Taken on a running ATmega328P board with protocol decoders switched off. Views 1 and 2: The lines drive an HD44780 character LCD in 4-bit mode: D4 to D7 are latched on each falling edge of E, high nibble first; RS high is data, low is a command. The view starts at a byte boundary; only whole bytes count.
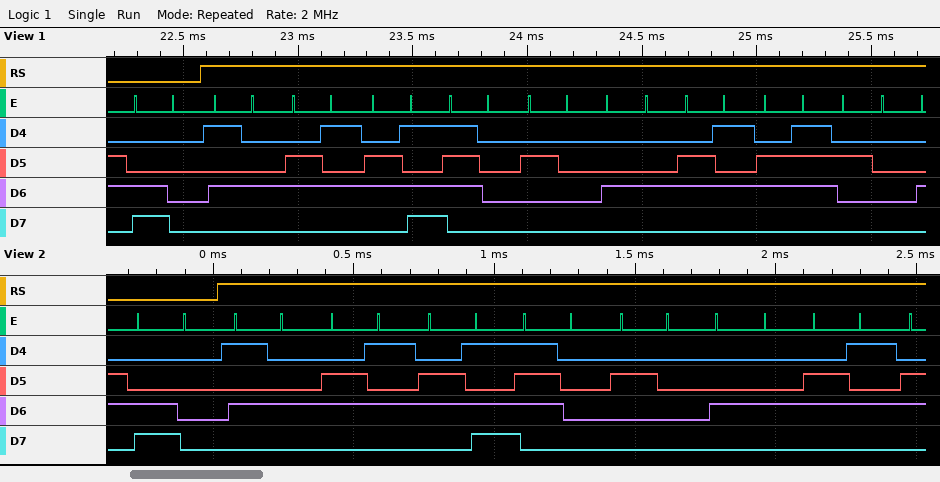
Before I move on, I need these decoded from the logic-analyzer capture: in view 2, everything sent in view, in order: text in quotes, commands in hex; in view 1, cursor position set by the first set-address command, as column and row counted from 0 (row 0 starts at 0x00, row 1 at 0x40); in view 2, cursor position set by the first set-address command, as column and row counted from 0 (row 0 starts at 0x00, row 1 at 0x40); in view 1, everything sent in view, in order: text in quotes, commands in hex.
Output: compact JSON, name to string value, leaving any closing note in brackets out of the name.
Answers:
{"in view 2, everything sent in view, in order: text in quotes, commands in hex": "0xC0 \"Temp De\"", "in view 1, cursor position set by the first set-address command, as column and row counted from 0": "column 0, row 1", "in view 2, cursor position set by the first set-address command, as column and row counted from 0": "column 0, row 1", "in view 1, everything sent in view, in order: text in quotes, commands in hex": "0xC0 \"Temp Deg \""}
